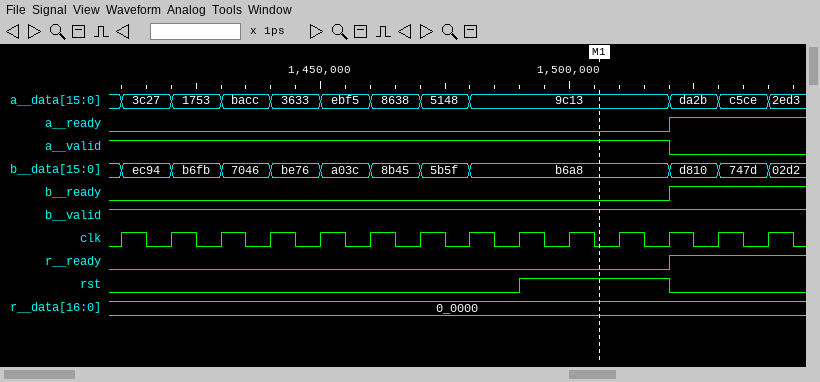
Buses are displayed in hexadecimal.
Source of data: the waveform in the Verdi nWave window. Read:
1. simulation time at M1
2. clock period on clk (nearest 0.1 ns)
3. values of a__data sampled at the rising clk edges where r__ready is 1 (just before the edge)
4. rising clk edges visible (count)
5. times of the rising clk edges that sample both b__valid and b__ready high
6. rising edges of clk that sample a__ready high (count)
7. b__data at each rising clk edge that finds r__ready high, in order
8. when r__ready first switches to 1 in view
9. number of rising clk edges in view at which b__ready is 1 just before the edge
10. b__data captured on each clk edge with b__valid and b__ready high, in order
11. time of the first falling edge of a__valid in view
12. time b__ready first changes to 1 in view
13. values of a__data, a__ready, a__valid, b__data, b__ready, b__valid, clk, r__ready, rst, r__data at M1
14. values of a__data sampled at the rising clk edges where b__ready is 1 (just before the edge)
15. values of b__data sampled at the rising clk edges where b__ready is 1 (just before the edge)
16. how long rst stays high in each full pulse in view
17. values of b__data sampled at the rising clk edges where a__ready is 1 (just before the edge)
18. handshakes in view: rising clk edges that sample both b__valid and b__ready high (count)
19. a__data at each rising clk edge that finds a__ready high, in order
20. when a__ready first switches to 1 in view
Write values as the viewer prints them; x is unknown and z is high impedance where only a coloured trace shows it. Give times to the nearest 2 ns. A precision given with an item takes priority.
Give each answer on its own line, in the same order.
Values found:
1506 ns
10 ns
da2b, c5ce
14
1530 ns, 1540 ns
2
d810, 747d
1520 ns
2
d810, 747d
1520 ns
1520 ns
a__data=9c13, a__ready=0, a__valid=1, b__data=b6a8, b__ready=0, b__valid=1, clk=0, r__ready=0, rst=1, r__data=0_0000
da2b, c5ce
d810, 747d
30 ns
d810, 747d
2
da2b, c5ce
1520 ns
